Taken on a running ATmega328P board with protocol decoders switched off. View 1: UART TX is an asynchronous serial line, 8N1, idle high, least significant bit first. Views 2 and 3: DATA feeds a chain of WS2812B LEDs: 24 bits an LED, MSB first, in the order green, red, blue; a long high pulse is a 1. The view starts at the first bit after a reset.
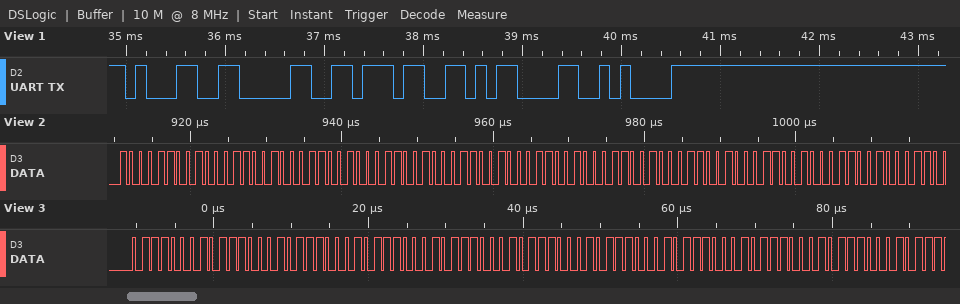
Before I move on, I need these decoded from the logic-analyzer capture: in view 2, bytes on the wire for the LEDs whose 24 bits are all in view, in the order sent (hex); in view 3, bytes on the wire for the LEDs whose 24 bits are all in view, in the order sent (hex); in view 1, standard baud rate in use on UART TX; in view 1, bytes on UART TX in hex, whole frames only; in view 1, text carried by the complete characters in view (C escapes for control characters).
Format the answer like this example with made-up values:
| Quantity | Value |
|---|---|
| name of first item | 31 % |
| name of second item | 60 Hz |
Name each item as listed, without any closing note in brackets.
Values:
| Quantity | Value |
|---|---|
| in view 2, bytes on the wire for the LEDs whose 24 bits are all in view, in the order sent | 8C 8C 8C 8C 8C 8C 8C 8C 8C |
| in view 3, bytes on the wire for the LEDs whose 24 bits are all in view, in the order sent | 71 71 71 71 71 71 71 71 71 |
| in view 1, standard baud rate in use on UART TX | 9600 baud |
| in view 1, bytes on UART TX in hex, whole frames only | 31 30 37 0D 0A |
| in view 1, text carried by the complete characters in view | "107\r\n" |
